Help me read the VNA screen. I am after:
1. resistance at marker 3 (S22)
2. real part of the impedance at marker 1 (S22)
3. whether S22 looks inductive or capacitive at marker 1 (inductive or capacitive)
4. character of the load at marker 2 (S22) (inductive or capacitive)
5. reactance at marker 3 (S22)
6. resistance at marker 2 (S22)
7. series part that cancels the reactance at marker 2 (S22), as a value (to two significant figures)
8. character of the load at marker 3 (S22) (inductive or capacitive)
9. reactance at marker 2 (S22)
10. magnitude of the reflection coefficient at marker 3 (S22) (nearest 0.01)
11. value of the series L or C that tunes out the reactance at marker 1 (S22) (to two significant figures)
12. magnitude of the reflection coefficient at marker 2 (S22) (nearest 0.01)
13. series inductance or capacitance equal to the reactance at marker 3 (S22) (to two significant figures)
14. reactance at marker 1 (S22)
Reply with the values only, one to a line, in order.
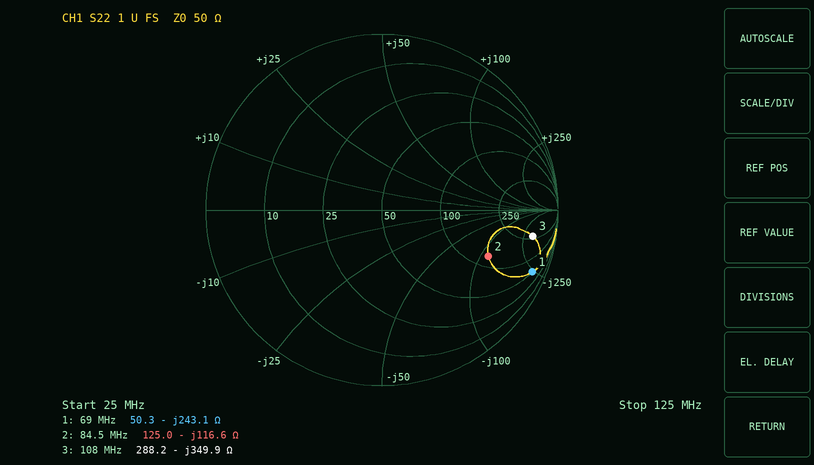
288.2 Ω
50.3 Ω
capacitive
capacitive
-349.9 Ω
125.0 Ω
220 nH
capacitive
-116.6 Ω
0.87
560 nH
0.66
4.2 pF
-243.1 Ω
